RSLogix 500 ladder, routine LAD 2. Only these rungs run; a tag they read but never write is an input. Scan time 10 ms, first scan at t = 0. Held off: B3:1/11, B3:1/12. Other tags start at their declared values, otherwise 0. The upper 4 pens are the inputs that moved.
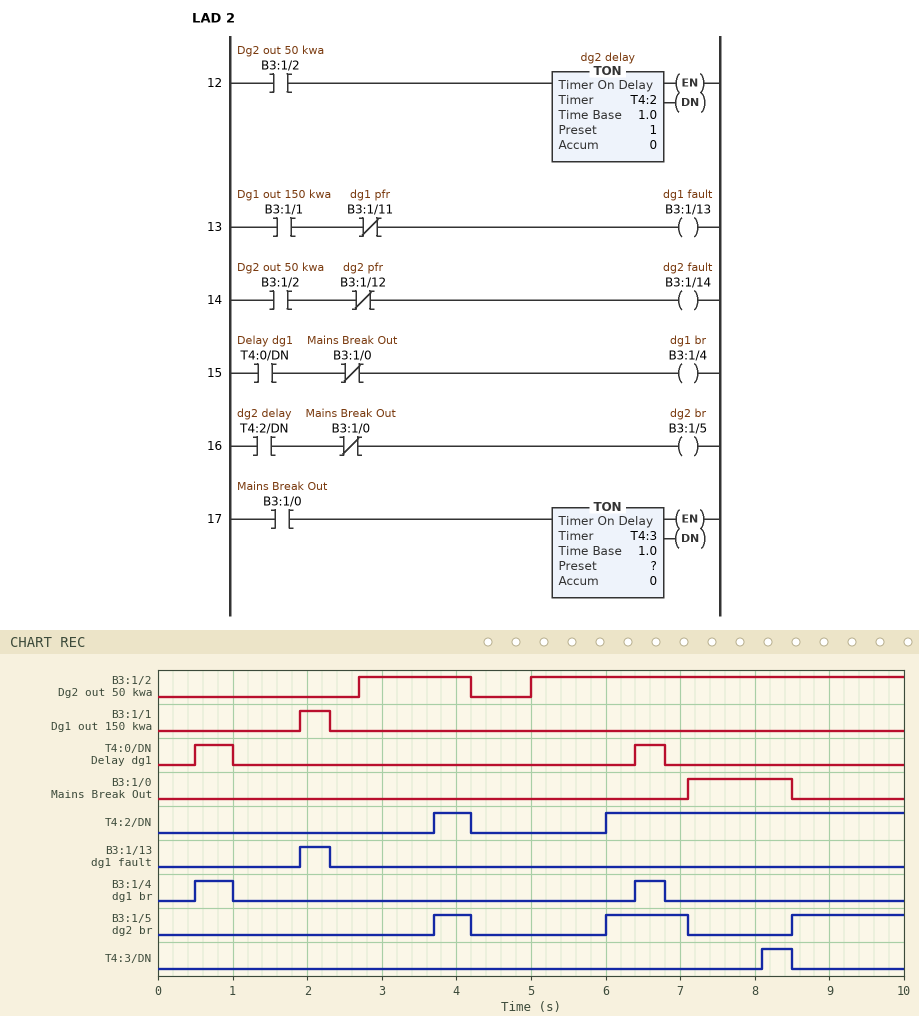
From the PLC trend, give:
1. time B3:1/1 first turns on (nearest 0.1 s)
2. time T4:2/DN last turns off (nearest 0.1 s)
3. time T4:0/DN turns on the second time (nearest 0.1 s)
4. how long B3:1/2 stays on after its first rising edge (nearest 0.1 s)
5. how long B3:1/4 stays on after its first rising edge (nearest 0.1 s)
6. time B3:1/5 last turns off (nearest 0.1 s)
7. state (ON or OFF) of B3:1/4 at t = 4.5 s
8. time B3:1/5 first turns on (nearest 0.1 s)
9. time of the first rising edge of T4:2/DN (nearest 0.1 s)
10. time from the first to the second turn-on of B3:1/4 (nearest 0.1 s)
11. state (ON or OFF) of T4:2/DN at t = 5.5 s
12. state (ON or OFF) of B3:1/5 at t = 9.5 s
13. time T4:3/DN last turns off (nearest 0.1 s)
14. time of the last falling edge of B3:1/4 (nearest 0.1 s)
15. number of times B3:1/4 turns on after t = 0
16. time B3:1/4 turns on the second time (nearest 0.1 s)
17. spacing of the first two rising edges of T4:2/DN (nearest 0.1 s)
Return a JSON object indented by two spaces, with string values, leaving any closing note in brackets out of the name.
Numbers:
{
  "time B3:1/1 first turns on": "1.9 s",
  "time T4:2/DN last turns off": "4.2 s",
  "time T4:0/DN turns on the second time": "6.4 s",
  "how long B3:1/2 stays on after its first rising edge": "1.5 s",
  "how long B3:1/4 stays on after its first rising edge": "0.5 s",
  "time B3:1/5 last turns off": "7.1 s",
  "state (ON or OFF) of B3:1/4 at t = 4.5 s": "OFF",
  "time B3:1/5 first turns on": "3.7 s",
  "time of the first rising edge of T4:2/DN": "3.7 s",
  "time from the first to the second turn-on of B3:1/4": "5.9 s",
  "state (ON or OFF) of T4:2/DN at t = 5.5 s": "OFF",
  "state (ON or OFF) of B3:1/5 at t = 9.5 s": "ON",
  "time T4:3/DN last turns off": "8.5 s",
  "time of the last falling edge of B3:1/4": "6.8 s",
  "number of times B3:1/4 turns on after t = 0": "2",
  "time B3:1/4 turns on the second time": "6.4 s",
  "spacing of the first two rising edges of T4:2/DN": "2.3 s"
}
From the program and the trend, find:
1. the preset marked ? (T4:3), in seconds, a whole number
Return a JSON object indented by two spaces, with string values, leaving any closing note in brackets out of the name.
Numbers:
{
  "the preset marked ? (T4:3), in seconds, a whole number": "1 s"
}
